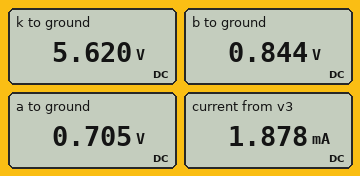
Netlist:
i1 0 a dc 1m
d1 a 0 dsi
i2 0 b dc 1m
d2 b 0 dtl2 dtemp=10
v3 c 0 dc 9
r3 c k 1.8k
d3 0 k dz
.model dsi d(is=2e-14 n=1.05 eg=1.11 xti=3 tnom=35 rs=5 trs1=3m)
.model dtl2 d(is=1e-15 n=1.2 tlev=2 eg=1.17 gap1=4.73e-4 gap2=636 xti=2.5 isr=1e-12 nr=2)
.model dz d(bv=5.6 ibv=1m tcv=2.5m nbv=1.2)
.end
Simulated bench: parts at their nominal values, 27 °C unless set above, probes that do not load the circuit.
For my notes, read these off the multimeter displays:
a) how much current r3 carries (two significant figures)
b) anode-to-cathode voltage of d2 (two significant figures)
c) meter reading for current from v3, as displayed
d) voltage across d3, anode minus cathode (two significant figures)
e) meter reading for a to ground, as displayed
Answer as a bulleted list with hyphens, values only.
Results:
- 1.9 mA
- 840 mV
- 1.878 mA
- -5.6 V
- 0.705 V
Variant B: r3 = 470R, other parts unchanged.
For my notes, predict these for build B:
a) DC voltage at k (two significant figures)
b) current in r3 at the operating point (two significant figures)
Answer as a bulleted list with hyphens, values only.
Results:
- 5.7 V
- 7.1 mA
